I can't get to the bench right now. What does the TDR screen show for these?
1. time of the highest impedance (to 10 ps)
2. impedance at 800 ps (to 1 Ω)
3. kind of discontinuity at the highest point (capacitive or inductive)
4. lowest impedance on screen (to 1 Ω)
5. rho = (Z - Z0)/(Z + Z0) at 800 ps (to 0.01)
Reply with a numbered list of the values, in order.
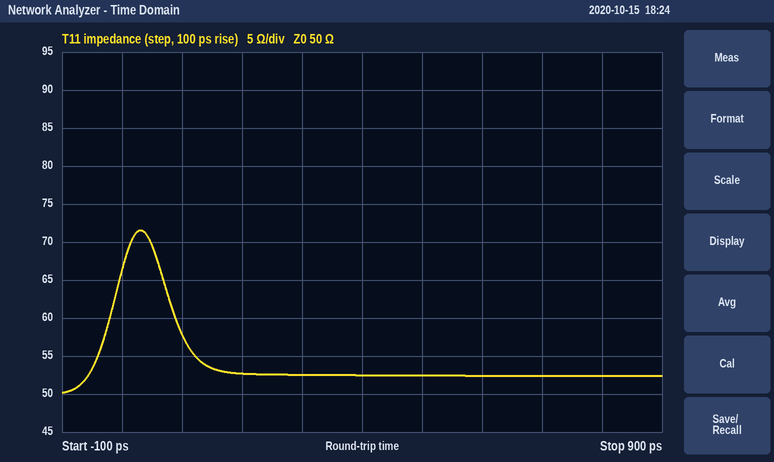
1. 30 ps
2. 52 Ω
3. inductive
4. 50 Ω
5. +0.02
